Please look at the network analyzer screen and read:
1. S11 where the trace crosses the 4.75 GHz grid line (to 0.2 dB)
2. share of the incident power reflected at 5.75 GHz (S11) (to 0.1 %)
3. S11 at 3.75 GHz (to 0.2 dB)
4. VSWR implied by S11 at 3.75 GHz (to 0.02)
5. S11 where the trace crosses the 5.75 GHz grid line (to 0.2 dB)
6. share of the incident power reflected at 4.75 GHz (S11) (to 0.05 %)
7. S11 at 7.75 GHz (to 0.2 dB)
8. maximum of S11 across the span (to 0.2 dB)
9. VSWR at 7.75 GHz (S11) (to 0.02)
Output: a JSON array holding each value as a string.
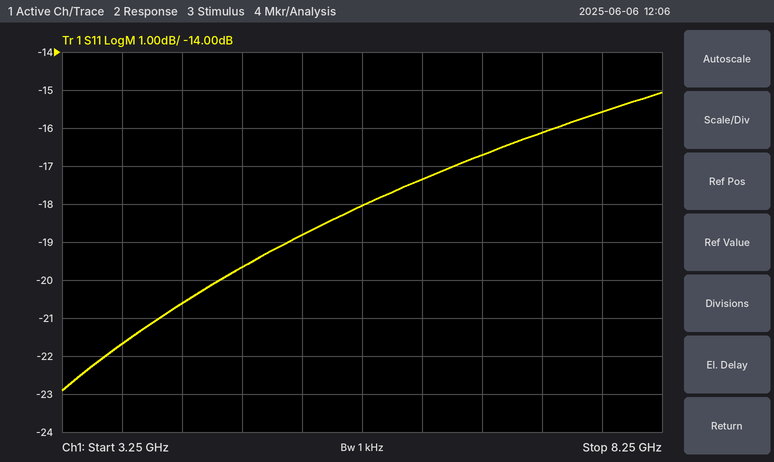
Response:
["-19.6 dB", "1.6 %", "-21.6 dB", "1.18", "-18.0 dB", "1.10 %", "-15.6 dB", "-15.0 dB", "1.40"]
